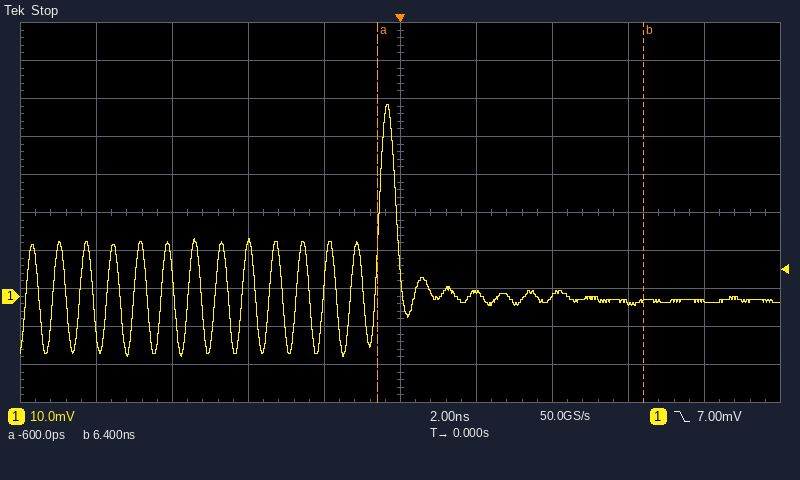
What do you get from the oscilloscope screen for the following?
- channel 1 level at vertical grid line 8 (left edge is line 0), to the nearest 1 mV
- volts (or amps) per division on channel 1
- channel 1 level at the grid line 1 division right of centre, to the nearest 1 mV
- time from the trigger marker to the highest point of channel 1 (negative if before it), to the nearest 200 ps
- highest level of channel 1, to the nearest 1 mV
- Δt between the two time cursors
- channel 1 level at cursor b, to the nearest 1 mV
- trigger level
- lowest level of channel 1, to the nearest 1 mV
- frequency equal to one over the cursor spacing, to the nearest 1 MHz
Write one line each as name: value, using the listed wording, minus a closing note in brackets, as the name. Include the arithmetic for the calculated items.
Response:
channel 1 level at vertical grid line 8 (left edge is line 0), to the nearest 1 mV: -2 mV
volts (or amps) per division on channel 1: 10 mV
channel 1 level at the grid line 1 division right of centre, to the nearest 1 mV: 1 mV
time from the trigger marker to the highest point of channel 1 (negative if before it), to the nearest 200 ps: -400 ps
highest level of channel 1, to the nearest 1 mV: 50 mV
Δt between the two time cursors: 6.4 ns − (-600 ps) = 7.0 ns
channel 1 level at cursor b, to the nearest 1 mV: -1 mV
trigger level: 7.00 mV
lowest level of channel 1, to the nearest 1 mV: -16 mV
frequency equal to one over the cursor spacing, to the nearest 1 MHz: 1 / 7.0 ns ≈ 143 MHz
